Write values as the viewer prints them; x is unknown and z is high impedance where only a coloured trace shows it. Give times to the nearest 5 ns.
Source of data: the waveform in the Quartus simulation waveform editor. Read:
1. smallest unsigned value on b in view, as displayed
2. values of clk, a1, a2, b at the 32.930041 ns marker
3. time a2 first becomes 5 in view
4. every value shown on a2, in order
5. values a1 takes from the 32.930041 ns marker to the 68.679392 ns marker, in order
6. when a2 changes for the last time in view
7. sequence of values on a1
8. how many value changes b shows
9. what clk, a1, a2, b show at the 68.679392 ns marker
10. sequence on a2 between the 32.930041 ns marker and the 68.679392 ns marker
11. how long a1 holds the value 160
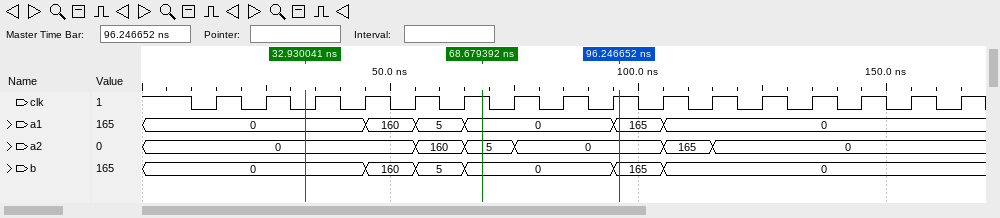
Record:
0
clk=0, a1=0, a2=0, b=0
65 ns
0, 160, 5, 0, 165, 0
0, 160, 5, 0
115 ns
0, 160, 5, 0, 165, 0
5
clk=1, a1=0, a2=5, b=0
0, 160, 5
10 ns
